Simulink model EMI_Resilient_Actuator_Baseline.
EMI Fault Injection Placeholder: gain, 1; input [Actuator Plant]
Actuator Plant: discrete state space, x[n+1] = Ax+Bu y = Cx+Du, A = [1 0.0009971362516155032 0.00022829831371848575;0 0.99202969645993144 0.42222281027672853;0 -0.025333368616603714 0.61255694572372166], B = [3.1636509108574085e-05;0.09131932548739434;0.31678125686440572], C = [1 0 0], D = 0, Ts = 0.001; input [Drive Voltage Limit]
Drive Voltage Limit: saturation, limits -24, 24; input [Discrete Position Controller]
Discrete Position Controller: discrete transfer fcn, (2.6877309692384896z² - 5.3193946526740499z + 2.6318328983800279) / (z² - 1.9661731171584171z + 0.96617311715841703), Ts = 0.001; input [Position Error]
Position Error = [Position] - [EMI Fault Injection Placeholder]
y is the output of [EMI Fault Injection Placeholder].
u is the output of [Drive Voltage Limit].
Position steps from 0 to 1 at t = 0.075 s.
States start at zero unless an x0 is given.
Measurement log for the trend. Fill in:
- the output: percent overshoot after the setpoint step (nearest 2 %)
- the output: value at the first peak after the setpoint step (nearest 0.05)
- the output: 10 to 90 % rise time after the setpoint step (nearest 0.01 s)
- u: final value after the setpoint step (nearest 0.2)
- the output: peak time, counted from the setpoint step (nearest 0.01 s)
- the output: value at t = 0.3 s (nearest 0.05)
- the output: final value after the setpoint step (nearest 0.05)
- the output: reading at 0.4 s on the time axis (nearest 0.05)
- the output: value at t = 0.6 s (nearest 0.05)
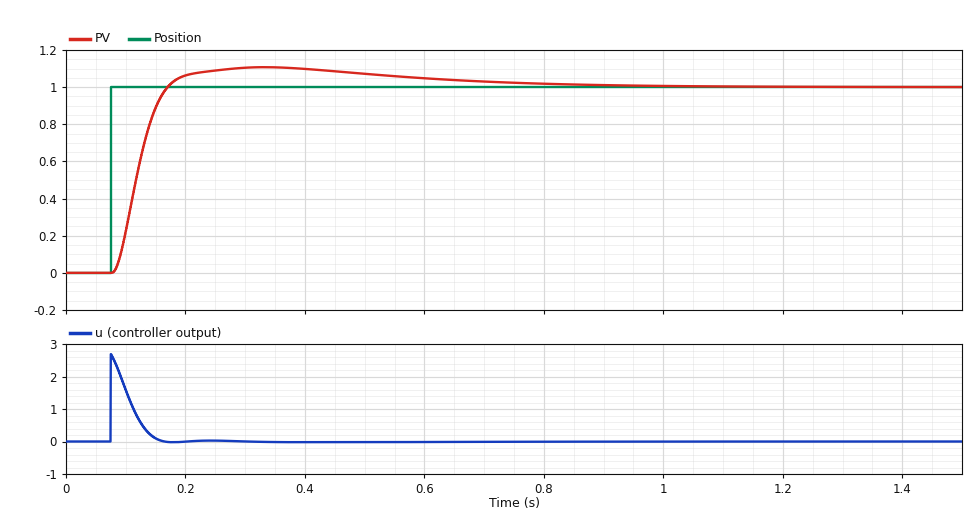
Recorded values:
10 %
1.10
0.06 s
0.0
0.26 s
1.10
1.00
1.10
1.05
